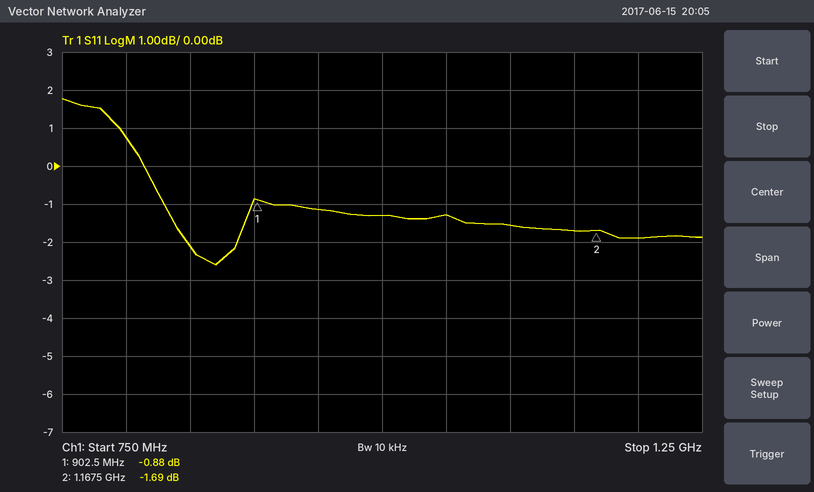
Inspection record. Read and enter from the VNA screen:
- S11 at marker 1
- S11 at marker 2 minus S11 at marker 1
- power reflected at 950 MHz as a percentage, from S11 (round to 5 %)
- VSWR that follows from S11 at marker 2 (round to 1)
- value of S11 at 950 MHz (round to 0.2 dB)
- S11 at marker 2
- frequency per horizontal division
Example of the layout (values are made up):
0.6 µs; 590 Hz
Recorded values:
-0.88 dB; -0.81 dB; 75 %; 10; -1.2 dB; -1.69 dB; 50 MHz
